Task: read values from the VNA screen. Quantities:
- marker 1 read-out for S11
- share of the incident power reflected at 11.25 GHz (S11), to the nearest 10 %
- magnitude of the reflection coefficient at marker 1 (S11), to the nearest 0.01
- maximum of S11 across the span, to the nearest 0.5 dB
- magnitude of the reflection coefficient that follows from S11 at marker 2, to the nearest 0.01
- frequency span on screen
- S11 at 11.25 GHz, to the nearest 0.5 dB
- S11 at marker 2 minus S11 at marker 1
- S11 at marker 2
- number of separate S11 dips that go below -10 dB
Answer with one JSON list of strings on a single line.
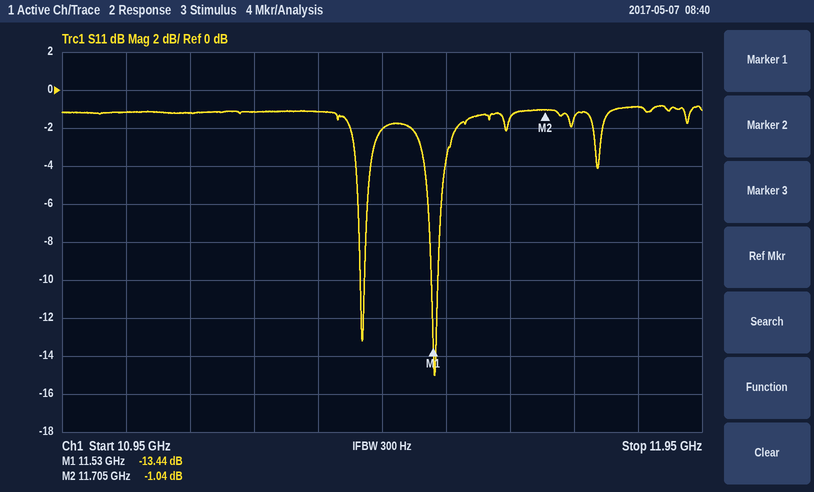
["-13.44 dB", "80 %", "0.21", "-1.0 dB", "0.89", "1 GHz", "-1.0 dB", "12.40 dB", "-1.04 dB", "2"]
